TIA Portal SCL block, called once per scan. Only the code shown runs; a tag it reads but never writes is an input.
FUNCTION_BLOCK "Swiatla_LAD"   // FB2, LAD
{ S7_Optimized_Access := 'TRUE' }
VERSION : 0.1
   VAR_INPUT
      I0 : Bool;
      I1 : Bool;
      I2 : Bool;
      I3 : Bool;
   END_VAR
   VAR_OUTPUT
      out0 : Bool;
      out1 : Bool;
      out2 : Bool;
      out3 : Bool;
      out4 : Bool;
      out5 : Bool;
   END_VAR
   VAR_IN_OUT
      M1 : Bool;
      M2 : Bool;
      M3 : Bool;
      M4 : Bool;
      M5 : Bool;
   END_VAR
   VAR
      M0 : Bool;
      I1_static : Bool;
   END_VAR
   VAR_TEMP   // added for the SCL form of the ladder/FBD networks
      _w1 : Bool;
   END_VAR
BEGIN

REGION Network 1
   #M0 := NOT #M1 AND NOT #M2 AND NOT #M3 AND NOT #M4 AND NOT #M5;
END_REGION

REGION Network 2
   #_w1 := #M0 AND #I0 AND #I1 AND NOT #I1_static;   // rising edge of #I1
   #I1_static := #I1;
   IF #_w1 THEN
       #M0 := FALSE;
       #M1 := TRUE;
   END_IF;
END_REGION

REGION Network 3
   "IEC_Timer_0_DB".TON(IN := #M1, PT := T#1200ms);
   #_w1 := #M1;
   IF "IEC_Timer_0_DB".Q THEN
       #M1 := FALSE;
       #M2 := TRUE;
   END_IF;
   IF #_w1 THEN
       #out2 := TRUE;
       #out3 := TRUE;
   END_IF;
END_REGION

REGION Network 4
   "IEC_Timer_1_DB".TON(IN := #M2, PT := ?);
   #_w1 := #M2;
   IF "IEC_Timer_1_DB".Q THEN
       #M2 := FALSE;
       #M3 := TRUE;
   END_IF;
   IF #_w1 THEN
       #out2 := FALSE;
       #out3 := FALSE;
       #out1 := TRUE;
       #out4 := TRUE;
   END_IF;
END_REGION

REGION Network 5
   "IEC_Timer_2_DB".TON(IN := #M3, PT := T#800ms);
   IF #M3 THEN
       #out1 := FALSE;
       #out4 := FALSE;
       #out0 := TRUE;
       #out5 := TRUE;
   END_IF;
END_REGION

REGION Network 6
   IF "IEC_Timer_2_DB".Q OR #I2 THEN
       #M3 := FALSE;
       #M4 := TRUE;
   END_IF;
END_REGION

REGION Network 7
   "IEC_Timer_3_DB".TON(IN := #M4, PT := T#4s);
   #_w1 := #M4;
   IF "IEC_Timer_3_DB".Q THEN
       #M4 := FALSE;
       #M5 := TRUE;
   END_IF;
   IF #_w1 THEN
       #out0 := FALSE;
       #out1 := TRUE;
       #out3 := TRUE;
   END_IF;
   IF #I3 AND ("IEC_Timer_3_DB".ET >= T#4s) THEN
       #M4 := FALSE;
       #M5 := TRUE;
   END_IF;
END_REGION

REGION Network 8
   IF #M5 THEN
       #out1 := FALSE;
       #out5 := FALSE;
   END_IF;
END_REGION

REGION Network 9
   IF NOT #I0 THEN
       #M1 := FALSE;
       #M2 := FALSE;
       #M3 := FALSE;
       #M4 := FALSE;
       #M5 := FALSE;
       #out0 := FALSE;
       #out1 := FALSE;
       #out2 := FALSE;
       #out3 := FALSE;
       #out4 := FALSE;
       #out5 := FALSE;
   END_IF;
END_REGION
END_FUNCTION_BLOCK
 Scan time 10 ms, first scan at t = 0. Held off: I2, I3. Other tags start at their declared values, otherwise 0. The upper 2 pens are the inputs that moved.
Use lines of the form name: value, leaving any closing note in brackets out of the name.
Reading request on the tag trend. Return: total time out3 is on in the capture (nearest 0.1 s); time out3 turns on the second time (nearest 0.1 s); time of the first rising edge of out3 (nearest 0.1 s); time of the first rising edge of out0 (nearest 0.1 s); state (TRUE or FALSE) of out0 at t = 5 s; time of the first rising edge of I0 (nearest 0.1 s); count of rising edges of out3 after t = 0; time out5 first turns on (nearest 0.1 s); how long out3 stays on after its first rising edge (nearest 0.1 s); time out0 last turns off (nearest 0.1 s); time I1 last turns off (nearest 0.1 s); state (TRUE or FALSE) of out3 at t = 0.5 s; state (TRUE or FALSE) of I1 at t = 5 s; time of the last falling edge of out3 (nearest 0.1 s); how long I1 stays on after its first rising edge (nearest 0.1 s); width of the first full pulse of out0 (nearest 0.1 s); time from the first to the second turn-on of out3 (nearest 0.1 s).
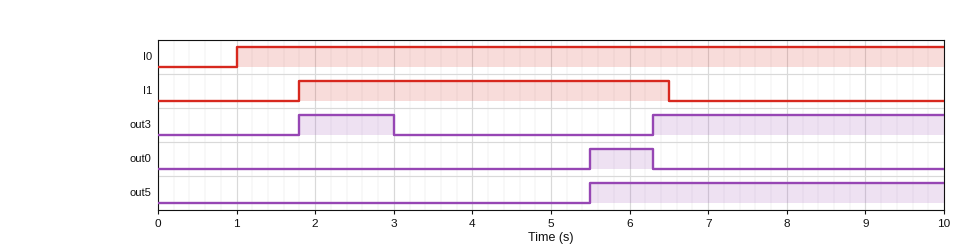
total time out3 is on in the capture: 4.9 s
time out3 turns on the second time: 6.3 s
time of the first rising edge of out3: 1.8 s
time of the first rising edge of out0: 5.5 s
state (TRUE or FALSE) of out0 at t = 5 s: FALSE
time of the first rising edge of I0: 1.0 s
count of rising edges of out3 after t = 0: 2
time out5 first turns on: 5.5 s
how long out3 stays on after its first rising edge: 1.2 s
time out0 last turns off: 6.3 s
time I1 last turns off: 6.5 s
state (TRUE or FALSE) of out3 at t = 0.5 s: FALSE
state (TRUE or FALSE) of I1 at t = 5 s: TRUE
time of the last falling edge of out3: 3.0 s
how long I1 stays on after its first rising edge: 4.7 s
width of the first full pulse of out0: 0.8 s
time from the first to the second turn-on of out3: 4.5 s
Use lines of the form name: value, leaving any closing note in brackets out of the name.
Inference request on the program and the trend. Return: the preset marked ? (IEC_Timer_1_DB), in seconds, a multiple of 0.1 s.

the preset marked ? (IEC_Timer_1_DB), in seconds, a multiple of 0.1 s: 2.5 s
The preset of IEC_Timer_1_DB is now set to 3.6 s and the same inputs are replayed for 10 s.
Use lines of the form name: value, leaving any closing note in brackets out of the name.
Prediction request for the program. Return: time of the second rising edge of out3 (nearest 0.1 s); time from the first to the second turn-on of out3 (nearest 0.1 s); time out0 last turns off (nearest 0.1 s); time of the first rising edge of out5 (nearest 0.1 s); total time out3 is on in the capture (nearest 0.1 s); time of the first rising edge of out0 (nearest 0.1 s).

time of the second rising edge of out3: 7.4 s
time from the first to the second turn-on of out3: 5.6 s
time out0 last turns off: 7.4 s
time of the first rising edge of out5: 6.6 s
total time out3 is on in the capture: 3.8 s
time of the first rising edge of out0: 6.6 s
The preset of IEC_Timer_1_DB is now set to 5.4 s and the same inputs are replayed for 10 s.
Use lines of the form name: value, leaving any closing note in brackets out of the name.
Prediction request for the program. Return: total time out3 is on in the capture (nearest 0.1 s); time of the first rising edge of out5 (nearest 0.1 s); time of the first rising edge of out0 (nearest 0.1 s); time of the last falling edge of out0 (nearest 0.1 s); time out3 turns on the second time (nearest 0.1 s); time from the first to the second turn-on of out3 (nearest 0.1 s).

total time out3 is on in the capture: 2.0 s
time of the first rising edge of out5: 8.4 s
time of the first rising edge of out0: 8.4 s
time of the last falling edge of out0: 9.2 s
time out3 turns on the second time: 9.2 s
time from the first to the second turn-on of out3: 7.4 s
